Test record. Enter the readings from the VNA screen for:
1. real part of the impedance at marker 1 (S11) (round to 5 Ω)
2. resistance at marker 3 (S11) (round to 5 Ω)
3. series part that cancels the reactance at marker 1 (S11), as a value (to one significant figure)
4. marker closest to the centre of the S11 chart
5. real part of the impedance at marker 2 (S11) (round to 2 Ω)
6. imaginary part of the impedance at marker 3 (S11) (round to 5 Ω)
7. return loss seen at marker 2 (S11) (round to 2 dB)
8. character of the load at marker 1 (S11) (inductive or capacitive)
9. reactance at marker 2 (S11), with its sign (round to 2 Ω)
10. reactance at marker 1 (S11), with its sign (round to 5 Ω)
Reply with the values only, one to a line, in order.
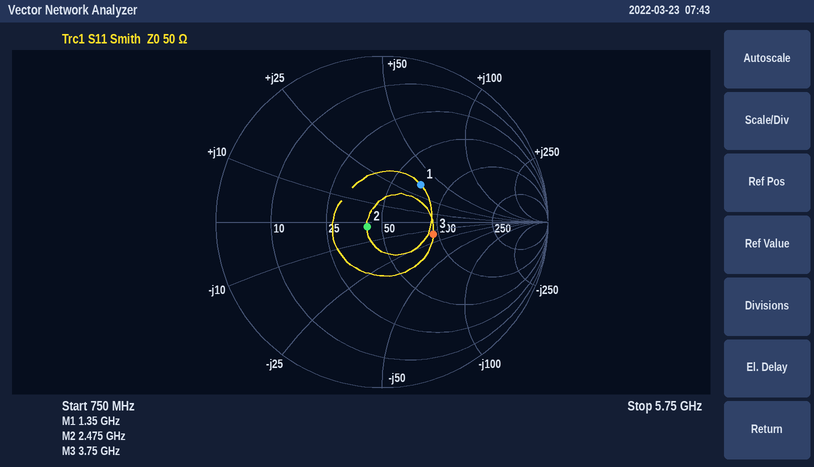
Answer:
70 Ω
95 Ω
3 pF
marker 2
42 Ω
-15 Ω
20 dB
inductive
-2 Ω
+35 Ω
